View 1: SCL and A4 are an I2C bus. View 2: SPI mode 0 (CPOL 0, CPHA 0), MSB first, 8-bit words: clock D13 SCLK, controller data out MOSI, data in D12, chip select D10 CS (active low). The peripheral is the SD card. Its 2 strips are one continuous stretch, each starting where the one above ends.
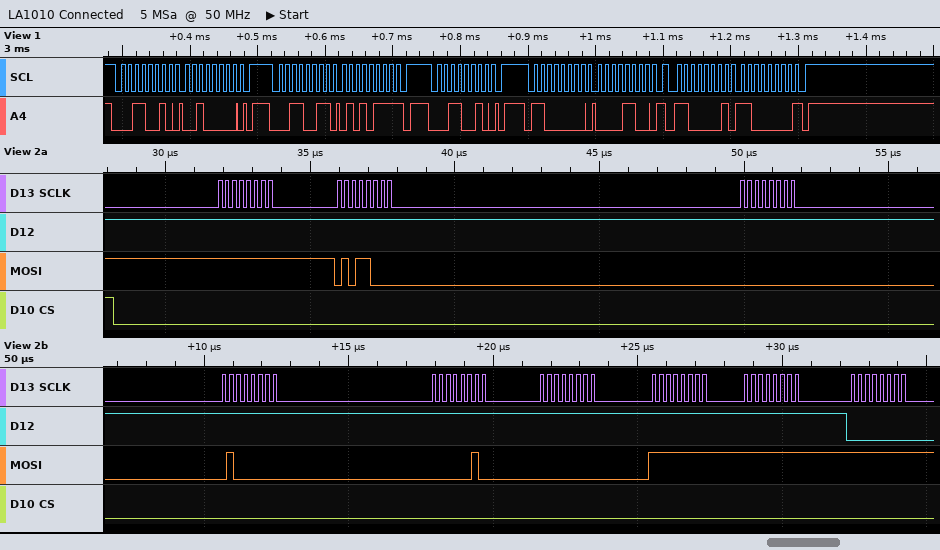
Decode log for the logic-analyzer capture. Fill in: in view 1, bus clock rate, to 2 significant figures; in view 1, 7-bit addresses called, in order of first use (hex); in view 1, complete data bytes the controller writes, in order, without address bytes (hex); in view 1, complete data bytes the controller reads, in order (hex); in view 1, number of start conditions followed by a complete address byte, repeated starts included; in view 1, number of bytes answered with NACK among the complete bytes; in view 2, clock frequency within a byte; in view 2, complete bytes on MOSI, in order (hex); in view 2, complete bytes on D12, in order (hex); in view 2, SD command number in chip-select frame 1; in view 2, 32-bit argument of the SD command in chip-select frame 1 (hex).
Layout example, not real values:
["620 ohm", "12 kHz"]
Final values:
["100 kHz", "0x19 0x60", "20 0C", "57 C0", "5", "2", "4 MHz", "0xFF 0x58 0x00 0x40 0x02 0x00 0xFF 0xFF 0xFF", "0xFF 0xFF 0xFF 0xFF 0xFF 0xFF 0xFF 0xFF 0x00", "CMD24", "0x00400200"]
